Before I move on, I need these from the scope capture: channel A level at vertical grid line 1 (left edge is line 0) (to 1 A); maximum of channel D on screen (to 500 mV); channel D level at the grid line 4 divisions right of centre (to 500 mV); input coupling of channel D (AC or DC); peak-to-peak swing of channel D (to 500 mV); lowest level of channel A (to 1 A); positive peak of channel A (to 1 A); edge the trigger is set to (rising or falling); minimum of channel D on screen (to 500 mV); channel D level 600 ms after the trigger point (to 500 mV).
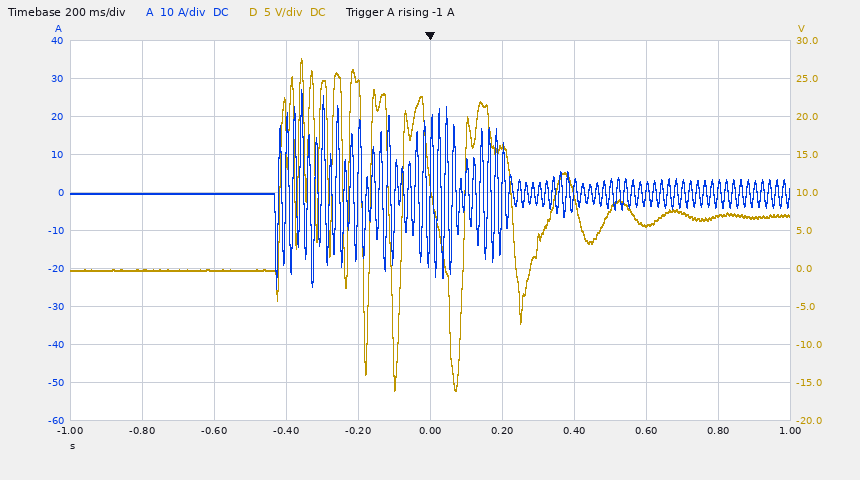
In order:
0 A
27.5 V
7.0 V
DC
43.5 V
-25 A
27 A
rising
-16.0 V
5.5 V
